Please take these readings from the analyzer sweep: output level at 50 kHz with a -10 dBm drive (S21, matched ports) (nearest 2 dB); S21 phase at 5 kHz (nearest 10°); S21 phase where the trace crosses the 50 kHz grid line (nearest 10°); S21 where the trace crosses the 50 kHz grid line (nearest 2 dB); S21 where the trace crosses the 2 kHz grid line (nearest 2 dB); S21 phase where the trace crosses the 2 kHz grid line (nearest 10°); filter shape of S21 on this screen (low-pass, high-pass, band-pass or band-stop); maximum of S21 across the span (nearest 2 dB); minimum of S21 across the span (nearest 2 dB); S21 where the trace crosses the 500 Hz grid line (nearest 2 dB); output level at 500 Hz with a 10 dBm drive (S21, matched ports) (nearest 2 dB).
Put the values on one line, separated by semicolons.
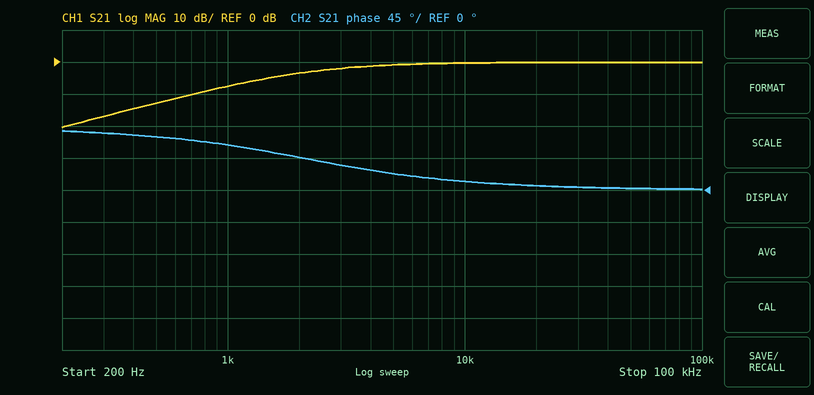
-10 dBm; 20°; 0°; 0 dB; -4 dB; 50°; high-pass; 0 dB; -20 dB; -12 dB; -2 dBm
